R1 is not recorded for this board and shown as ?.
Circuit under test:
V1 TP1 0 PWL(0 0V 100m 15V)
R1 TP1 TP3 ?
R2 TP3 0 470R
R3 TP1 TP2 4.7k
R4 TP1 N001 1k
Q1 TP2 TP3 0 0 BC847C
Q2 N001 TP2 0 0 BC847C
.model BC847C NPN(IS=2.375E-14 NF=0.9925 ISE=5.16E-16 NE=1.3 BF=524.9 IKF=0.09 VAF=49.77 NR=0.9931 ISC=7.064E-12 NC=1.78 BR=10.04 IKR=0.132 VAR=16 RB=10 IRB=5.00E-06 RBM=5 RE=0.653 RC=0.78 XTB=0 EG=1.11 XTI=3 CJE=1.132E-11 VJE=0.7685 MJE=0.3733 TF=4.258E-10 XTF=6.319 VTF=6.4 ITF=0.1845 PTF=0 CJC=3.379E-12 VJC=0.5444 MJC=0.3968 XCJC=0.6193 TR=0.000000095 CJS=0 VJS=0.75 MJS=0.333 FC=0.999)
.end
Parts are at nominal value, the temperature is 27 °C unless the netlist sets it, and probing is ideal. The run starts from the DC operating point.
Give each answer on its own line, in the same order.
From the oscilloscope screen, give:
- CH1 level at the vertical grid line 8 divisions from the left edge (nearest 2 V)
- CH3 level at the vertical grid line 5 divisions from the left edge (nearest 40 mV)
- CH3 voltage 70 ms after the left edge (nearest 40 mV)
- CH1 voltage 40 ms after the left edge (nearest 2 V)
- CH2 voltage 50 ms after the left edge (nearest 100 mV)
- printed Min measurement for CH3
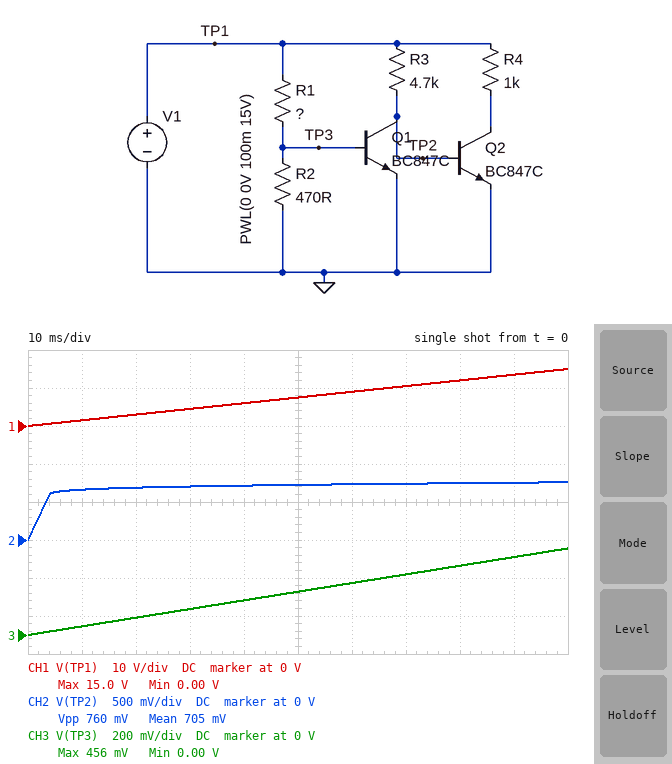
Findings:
12 V
240 mV
320 mV
6 V
700 mV
0.00 V
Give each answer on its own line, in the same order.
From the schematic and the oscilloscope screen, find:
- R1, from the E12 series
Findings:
15 kΩ
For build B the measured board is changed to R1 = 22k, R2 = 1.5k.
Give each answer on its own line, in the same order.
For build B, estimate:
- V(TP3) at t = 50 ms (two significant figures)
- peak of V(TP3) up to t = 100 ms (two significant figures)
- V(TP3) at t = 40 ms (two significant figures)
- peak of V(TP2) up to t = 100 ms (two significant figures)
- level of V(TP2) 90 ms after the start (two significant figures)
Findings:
480 mV
680 mV
380 mV
730 mV
38 mV
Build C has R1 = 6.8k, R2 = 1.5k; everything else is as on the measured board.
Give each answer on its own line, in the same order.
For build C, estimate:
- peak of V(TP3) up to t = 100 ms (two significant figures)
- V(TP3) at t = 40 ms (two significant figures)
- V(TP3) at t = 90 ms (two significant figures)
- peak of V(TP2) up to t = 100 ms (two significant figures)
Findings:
720 mV
670 mV
710 mV
690 mV
